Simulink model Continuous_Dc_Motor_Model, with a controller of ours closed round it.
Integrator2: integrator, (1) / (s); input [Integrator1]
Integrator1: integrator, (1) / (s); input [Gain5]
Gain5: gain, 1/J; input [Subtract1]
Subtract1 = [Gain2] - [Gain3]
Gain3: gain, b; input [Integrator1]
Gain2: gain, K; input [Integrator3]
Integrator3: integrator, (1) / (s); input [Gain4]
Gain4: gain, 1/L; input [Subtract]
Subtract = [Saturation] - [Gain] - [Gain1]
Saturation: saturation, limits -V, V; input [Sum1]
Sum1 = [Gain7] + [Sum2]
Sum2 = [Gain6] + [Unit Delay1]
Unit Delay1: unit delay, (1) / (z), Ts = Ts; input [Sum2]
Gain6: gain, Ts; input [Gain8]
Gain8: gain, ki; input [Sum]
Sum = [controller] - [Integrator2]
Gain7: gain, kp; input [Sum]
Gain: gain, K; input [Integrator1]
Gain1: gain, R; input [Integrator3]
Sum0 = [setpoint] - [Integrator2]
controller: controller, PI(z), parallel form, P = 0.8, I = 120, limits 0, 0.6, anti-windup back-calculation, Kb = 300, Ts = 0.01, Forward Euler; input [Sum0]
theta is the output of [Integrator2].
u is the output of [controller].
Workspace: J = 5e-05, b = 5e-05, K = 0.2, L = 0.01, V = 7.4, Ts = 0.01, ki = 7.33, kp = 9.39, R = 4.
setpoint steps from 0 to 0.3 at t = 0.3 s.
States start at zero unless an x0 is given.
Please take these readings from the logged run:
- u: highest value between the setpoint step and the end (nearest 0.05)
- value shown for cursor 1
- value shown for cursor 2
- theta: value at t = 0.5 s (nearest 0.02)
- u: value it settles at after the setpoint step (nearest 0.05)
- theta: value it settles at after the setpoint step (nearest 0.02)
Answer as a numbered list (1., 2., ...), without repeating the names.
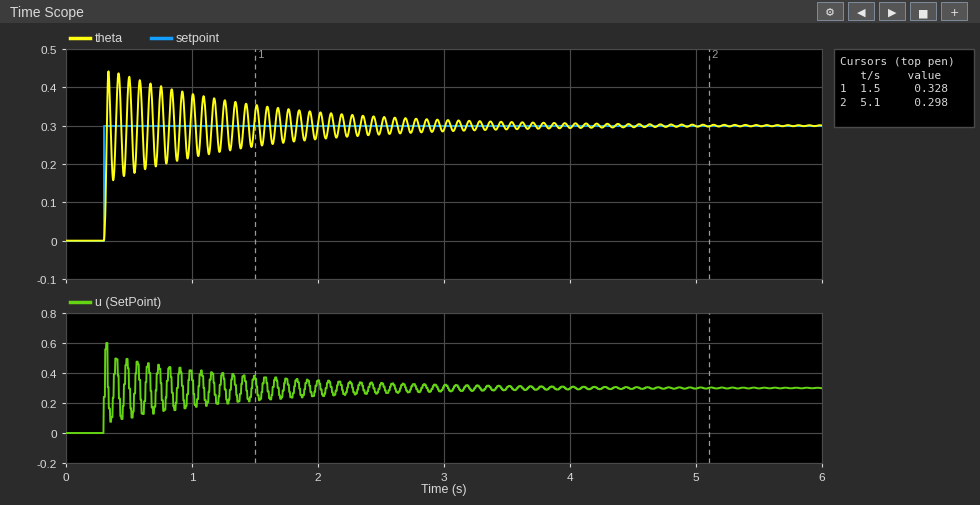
1. 0.60
2. 0.328
3. 0.298
4. 0.42
5. 0.30
6. 0.30
